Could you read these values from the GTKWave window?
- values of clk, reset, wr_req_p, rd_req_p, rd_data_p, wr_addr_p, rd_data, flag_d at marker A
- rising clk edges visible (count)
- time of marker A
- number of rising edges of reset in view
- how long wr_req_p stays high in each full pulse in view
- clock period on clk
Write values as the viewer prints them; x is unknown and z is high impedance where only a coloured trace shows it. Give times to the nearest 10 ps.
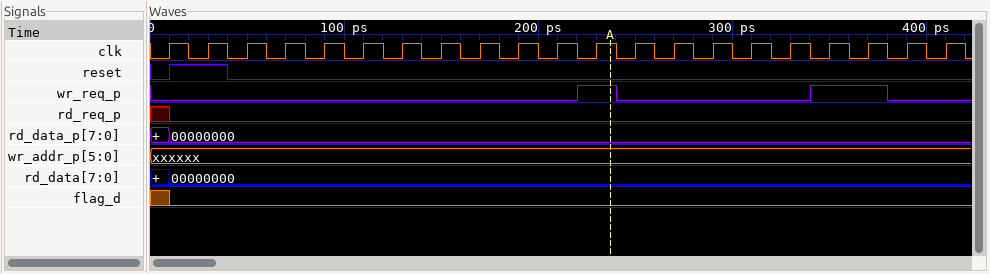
clk=1, reset=0, wr_req_p=1, rd_req_p=0, rd_data_p=00000000, wr_addr_p=xxxxxx, rd_data=00000000, flag_d=0
21
240 ps
1
20 ps, 40 ps
20 ps
